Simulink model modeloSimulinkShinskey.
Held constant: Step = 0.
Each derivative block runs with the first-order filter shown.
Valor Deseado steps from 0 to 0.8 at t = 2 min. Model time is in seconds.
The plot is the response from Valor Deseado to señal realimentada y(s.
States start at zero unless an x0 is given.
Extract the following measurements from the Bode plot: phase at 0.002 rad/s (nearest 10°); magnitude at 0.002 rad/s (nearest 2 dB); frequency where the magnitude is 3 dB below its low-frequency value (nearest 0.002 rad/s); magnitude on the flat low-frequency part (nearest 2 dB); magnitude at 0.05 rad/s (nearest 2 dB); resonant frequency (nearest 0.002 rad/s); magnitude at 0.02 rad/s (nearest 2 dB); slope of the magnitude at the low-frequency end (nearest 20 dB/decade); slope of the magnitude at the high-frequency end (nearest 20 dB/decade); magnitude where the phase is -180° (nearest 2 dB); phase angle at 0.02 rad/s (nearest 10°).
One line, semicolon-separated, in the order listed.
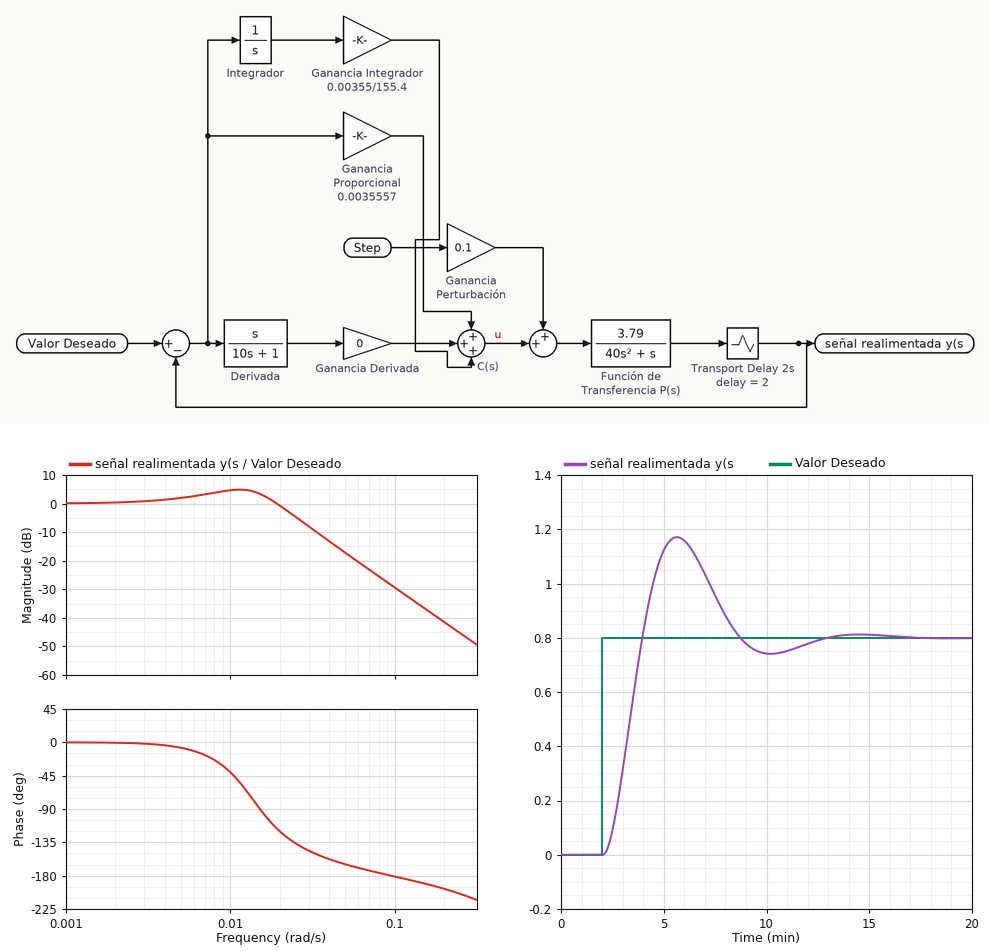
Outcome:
0°; 0 dB; 0.022 rad/s; 0 dB; -18 dB; 0.012 rad/s; 0 dB; 0 dB/decade; -40 dB/decade; -28 dB; -120°
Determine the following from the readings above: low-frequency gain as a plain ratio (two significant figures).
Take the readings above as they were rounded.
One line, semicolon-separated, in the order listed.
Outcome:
1.0
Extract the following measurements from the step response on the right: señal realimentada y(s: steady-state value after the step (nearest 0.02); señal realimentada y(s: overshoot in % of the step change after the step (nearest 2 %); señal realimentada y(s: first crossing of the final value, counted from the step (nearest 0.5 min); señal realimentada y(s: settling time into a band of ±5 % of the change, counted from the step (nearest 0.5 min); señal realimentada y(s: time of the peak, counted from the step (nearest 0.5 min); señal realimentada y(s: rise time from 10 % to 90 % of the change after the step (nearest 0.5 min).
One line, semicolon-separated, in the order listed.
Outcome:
0.80; 46 %; 2.0 min; 9.5 min; 3.5 min; 1.5 min
